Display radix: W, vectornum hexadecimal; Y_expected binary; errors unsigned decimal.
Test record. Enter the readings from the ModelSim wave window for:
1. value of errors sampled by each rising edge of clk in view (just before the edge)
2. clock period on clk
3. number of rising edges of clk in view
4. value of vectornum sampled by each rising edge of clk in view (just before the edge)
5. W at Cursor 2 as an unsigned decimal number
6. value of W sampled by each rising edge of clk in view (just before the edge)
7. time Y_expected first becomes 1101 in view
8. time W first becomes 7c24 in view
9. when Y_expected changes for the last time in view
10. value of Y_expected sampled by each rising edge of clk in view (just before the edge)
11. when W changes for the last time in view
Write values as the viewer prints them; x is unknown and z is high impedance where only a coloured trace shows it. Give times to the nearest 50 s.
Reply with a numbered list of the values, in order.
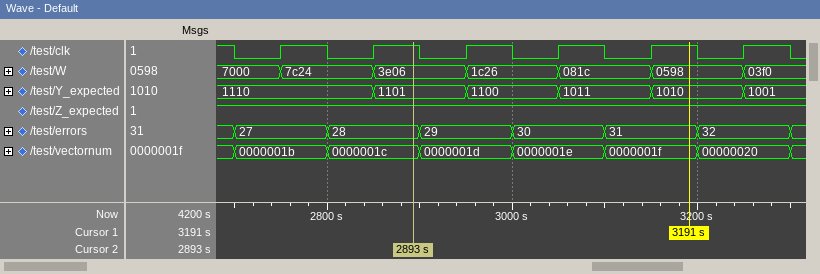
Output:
1. 27, 28, 29, 30, 31, 32
2. 100 s
3. 6
4. 0000001b, 0000001c, 0000001d, 0000001e, 0000001f, 00000020
5. 15878
6. 7000, 7c24, 3e06, 1c26, 081c, 0598
7. 2850 s
8. 2750 s
9. 3250 s
10. 1110, 1110, 1101, 1100, 1011, 1010
11. 3250 s
